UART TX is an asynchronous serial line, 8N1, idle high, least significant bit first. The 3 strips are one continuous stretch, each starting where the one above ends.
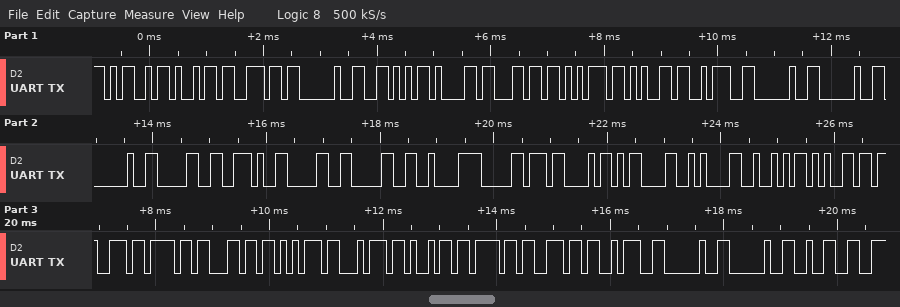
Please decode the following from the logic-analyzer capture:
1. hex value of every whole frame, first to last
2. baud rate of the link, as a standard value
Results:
0x4D 0x69 0x6E 0x20 0x56 0x61 0x6C 0x75 0x65 0x3A 0x20 0x20 0x20 0x30 0x2E 0x30 0x30 0xC2 0xB0 0x43 0x0D 0x0A 0x52 0x65 0x73 0x6F 0x6C 0x75 0x74 0x69 0x6F 0x6E 0x3A 0x20 0x20 0x32
9600 baud
